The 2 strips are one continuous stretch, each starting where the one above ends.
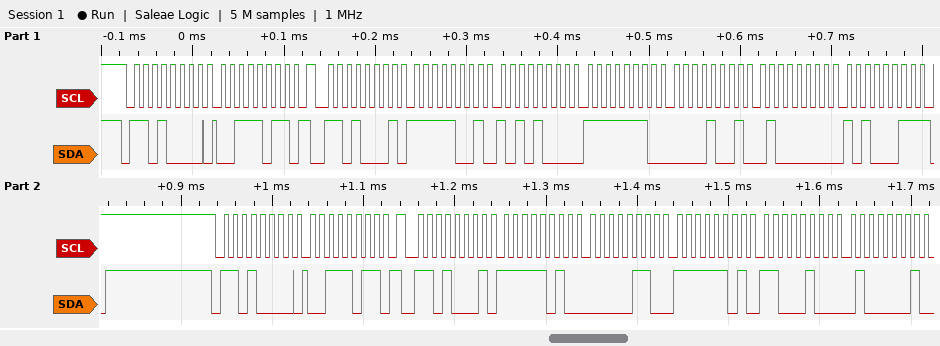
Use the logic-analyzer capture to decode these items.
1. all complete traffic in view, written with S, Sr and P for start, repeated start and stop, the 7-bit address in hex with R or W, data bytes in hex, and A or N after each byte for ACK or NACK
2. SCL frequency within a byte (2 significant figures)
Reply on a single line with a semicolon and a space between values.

S 68W A 3B A Sr 68R A F9 A A8 A FE A 09 A 40 A A3 N P S 68W A 3B A Sr 68R A FA A 06 A FD A C4 A 41 A; 100 kHz
